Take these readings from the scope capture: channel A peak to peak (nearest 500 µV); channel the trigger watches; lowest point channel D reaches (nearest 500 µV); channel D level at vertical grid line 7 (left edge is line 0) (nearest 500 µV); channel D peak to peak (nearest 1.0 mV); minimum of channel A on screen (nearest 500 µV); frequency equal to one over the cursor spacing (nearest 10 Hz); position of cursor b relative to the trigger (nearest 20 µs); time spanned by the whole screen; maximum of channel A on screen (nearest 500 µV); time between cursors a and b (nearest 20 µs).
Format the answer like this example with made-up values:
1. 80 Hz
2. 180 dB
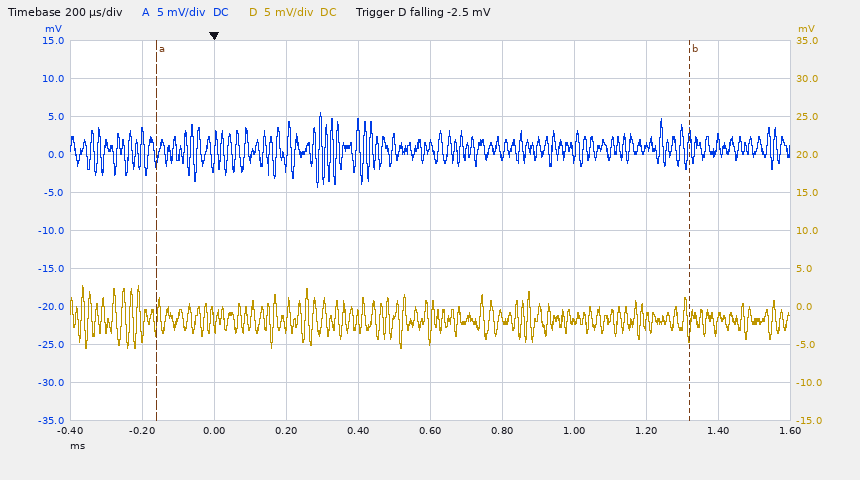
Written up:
1. 10.0 mV
2. channel D
3. -5.5 mV
4. -2.0 mV
5. 8.0 mV
6. -4.5 mV
7. 680 Hz
8. +1.32 ms
9. 2 ms
10. 5.5 mV
11. 1.48 ms
